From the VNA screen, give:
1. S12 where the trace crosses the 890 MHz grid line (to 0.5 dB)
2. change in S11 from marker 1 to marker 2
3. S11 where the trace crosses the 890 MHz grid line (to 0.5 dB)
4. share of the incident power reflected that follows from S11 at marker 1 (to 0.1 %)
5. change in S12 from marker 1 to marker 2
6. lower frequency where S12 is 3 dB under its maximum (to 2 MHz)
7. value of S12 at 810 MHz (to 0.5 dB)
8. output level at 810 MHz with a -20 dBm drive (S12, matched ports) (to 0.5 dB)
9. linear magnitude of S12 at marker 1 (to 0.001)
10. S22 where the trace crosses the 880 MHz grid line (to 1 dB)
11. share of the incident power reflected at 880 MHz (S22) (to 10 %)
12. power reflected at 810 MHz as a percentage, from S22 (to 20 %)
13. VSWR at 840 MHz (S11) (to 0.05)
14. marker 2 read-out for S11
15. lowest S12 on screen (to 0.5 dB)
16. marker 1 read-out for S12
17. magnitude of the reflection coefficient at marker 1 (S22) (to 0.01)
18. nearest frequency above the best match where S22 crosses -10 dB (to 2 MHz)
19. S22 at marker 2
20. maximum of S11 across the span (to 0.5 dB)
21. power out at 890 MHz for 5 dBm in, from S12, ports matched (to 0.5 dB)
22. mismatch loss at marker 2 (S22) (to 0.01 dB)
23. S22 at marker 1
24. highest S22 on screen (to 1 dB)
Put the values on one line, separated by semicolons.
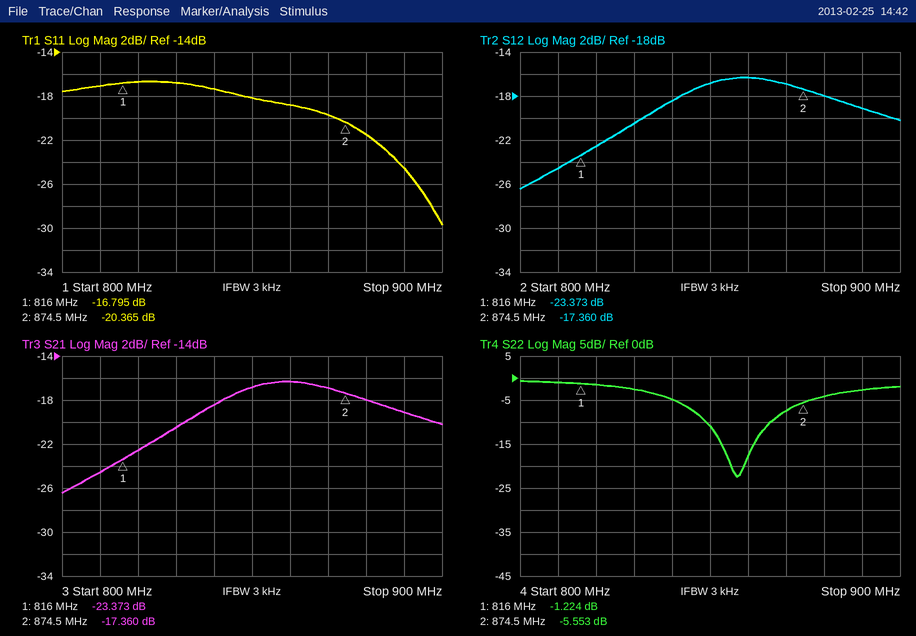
-19.0 dB; -3.570 dB; -24.5 dB; 2.1 %; 6.013 dB; 836 MHz; -24.5 dB; -44.5 dBm; 0.068; -4 dB; 40 %; 80 %; 1.30; -20.365 dB; -26.5 dB; -23.373 dB; 0.87; 866 MHz; -5.553 dB; -16.5 dB; -14.0 dBm; 1.42 dB; -1.224 dB; -1 dB
